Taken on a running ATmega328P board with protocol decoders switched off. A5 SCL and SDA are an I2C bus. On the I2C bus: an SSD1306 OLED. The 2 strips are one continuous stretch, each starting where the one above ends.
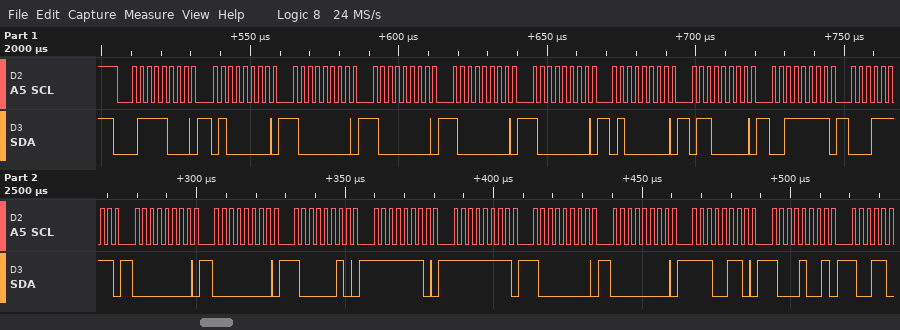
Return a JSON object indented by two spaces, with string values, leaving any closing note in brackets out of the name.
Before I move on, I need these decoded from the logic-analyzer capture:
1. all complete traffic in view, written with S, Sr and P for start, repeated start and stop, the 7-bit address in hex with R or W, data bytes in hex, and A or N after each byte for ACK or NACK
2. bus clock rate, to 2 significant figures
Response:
{
  "all complete traffic in view, written with S, Sr and P for start, repeated start and stop, the 7-bit address in hex with R or W, data bytes in hex, and A or N after each byte for ACK or NACK": "S 3CW A 40 A 80 A 80 A 80 A 80 A 40 A 60 A 3F A 1F A 00 A 00 A 82 A FE A FF A 80 A 00 A E6 A 89 A",
  "bus clock rate, to 2 significant figures": "400 kHz"
}
